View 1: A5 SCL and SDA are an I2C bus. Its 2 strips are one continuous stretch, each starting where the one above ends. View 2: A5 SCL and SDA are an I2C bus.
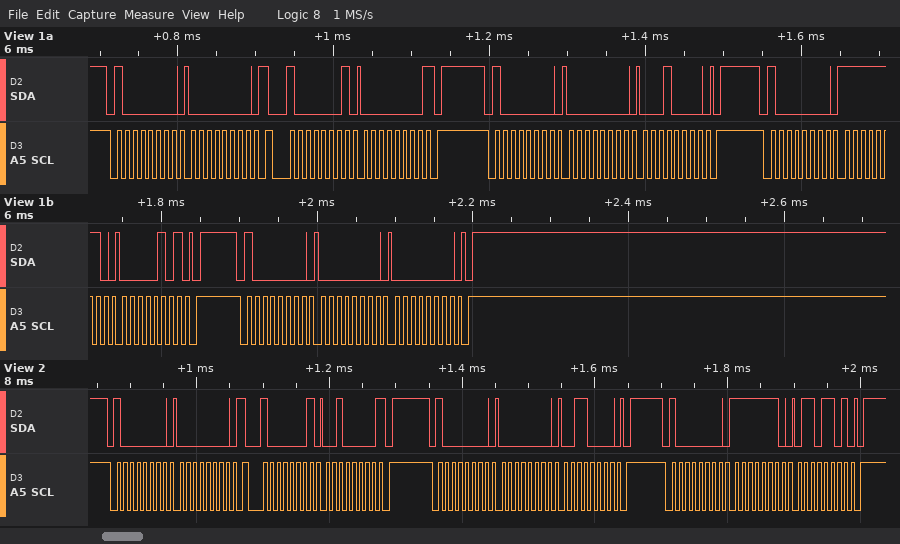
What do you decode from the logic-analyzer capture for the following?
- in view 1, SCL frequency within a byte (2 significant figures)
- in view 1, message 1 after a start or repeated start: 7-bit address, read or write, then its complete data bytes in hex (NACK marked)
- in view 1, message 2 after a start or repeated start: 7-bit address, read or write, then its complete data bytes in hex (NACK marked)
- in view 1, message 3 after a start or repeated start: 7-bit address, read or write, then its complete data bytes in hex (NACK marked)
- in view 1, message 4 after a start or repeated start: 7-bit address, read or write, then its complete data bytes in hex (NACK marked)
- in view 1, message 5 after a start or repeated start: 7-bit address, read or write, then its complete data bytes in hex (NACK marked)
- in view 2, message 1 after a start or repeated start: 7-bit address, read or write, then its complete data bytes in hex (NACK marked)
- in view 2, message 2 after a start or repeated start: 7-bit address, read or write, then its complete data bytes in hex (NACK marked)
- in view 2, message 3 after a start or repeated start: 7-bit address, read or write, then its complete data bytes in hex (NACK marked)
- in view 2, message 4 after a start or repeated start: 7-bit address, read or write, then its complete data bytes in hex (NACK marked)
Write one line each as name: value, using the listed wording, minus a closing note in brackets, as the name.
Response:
in view 1, SCL frequency within a byte: 100 kHz
in view 1, message 1 after a start or repeated start: 7-bit address, read or write, then its complete data bytes in hex: 0x40 write: 00
in view 1, message 2 after a start or repeated start: 7-bit address, read or write, then its complete data bytes in hex: 0x40 read: 00 NACK
in view 1, message 3 after a start or repeated start: 7-bit address, read or write, then its complete data bytes in hex: 0x40 write: 00 10
in view 1, message 4 after a start or repeated start: 7-bit address, read or write, then its complete data bytes in hex: 0x40 write: FE 05
in view 1, message 5 after a start or repeated start: 7-bit address, read or write, then its complete data bytes in hex: 0x40 write: 00 00
in view 2, message 1 after a start or repeated start: 7-bit address, read or write, then its complete data bytes in hex: 0x40 write: 00
in view 2, message 2 after a start or repeated start: 7-bit address, read or write, then its complete data bytes in hex: 0x40 read: 20 NACK
in view 2, message 3 after a start or repeated start: 7-bit address, read or write, then its complete data bytes in hex: 0x40 write: 00 30
in view 2, message 4 after a start or repeated start: 7-bit address, read or write, then its complete data bytes in hex: 0x40 write: FE 6D
